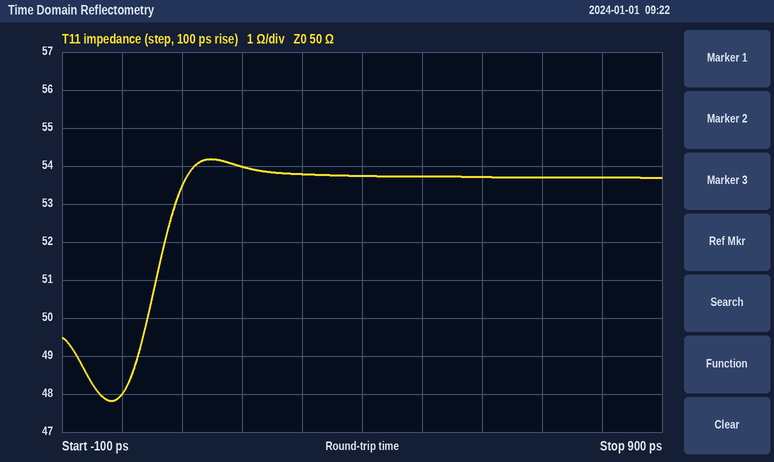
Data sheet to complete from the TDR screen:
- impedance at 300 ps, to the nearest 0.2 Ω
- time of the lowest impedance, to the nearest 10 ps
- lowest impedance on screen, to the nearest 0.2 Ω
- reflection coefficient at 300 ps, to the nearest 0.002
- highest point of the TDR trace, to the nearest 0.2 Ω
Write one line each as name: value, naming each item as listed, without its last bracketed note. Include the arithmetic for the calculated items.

impedance at 300 ps, to the nearest 0.2 Ω: 53.8 Ω
time of the lowest impedance, to the nearest 10 ps: -20 ps
lowest impedance on screen, to the nearest 0.2 Ω: 47.8 Ω
reflection coefficient at 300 ps, to the nearest 0.002: (53.8 − 50)/(53.8 + 50) ≈ +0.0366, so +0.036 to the nearest 0.002
highest point of the TDR trace, to the nearest 0.2 Ω: 54.2 Ω
